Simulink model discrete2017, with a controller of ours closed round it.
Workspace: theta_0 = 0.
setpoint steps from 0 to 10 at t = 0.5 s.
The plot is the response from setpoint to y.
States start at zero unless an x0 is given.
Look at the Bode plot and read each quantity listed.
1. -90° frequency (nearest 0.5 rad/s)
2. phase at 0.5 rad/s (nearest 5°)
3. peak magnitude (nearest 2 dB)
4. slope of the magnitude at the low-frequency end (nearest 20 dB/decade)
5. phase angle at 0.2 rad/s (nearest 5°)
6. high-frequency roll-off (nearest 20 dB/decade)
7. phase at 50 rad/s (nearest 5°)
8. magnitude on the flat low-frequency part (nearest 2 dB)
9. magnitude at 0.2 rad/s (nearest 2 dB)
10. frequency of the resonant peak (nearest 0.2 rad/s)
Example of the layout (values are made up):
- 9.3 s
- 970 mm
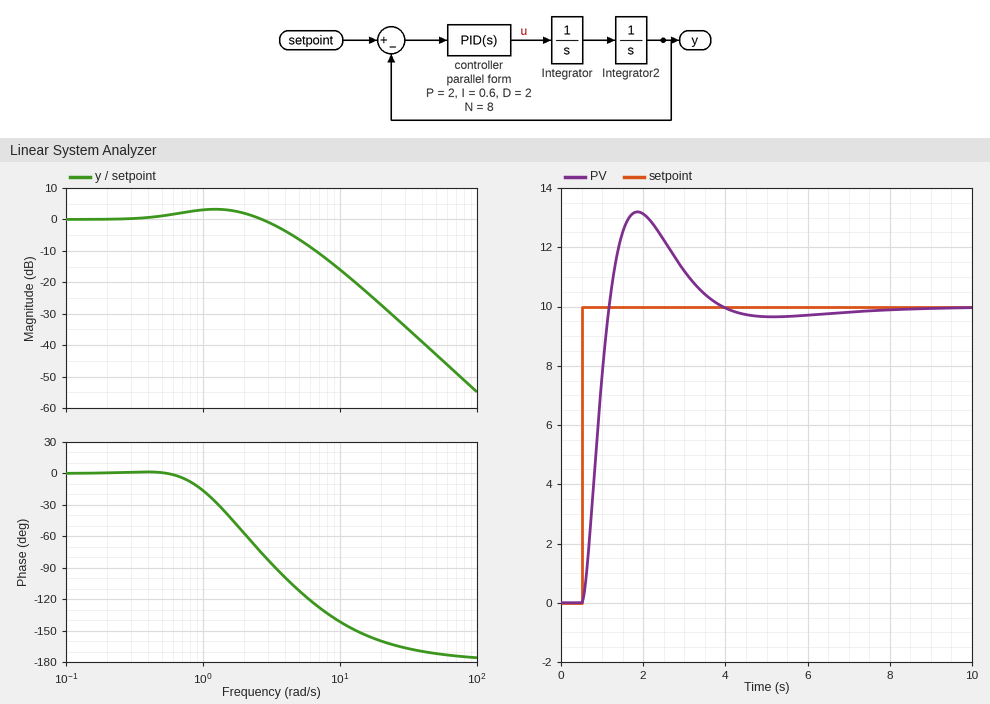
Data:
- 3.5 rad/s
- 0°
- 4 dB
- 0 dB/decade
- 0°
- -40 dB/decade
- -170°
- 0 dB
- 0 dB
- 1.2 rad/s
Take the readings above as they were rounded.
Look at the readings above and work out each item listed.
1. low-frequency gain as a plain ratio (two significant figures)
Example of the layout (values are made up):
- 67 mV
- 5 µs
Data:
- 1.0
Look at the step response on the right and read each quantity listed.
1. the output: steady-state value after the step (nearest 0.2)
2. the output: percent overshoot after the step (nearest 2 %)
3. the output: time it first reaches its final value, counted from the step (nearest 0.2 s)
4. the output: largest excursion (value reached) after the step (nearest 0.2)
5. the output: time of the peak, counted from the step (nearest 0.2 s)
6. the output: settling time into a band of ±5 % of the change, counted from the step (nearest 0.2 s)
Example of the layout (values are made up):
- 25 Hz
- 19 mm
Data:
- 10.0
- 32 %
- 0.6 s
- 13.2
- 1.4 s
- 3.0 s
